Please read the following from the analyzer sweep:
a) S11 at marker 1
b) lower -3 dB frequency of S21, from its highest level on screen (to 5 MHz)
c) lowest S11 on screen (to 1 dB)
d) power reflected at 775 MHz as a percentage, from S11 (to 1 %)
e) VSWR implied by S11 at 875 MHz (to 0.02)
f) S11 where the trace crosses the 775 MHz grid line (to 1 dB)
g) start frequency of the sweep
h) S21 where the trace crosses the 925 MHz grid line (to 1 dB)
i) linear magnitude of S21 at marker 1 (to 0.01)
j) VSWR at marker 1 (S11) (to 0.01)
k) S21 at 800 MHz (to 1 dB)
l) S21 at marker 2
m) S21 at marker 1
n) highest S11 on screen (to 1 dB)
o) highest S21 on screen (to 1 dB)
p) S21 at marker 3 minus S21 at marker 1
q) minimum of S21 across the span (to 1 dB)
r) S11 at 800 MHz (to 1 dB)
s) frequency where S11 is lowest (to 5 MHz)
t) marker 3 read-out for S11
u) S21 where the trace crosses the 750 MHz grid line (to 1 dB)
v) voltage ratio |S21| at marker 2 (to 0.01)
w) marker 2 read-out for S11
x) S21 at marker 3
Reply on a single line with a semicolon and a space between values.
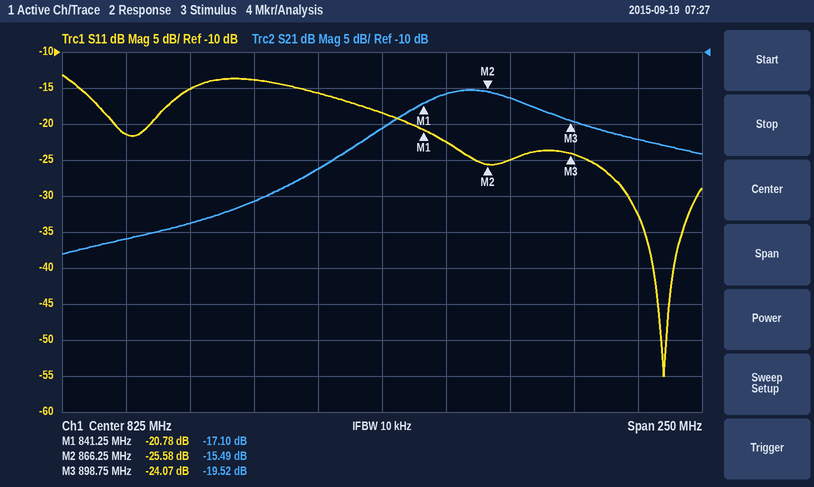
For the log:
-20.78 dB; 835 MHz; -55 dB; 4 %; 1.12; -14 dB; 700 MHz; -22 dB; 0.14; 1.20; -26 dB; -15.49 dB; -17.10 dB; -13 dB; -15 dB; -2.42 dB; -38 dB; -16 dB; 935 MHz; -24.07 dB; -34 dB; 0.17; -25.58 dB; -19.52 dB
